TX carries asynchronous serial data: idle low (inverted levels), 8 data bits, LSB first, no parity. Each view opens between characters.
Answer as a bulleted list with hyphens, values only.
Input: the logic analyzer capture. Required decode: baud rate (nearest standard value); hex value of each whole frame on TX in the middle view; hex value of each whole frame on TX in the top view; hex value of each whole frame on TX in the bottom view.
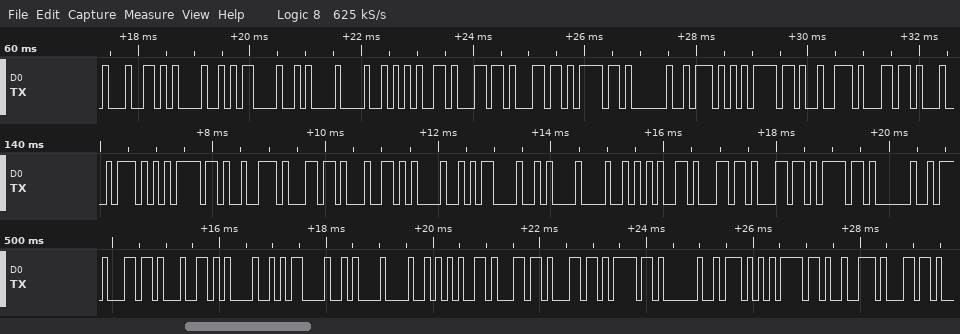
- 9600 baud
- 51, 21, 1B, 27, 37, BD, E5, EB, 6F, 35, 27, 27, 21, BF
- 37, BD, E5, EB, 6F, 35, 27, 27, 21, BF, 51, 21, 1B, 27
- 27, 37, BD, E5, EB, 6F, 35, 27, 27, 21, BF, 51, 21, 1B, 27
